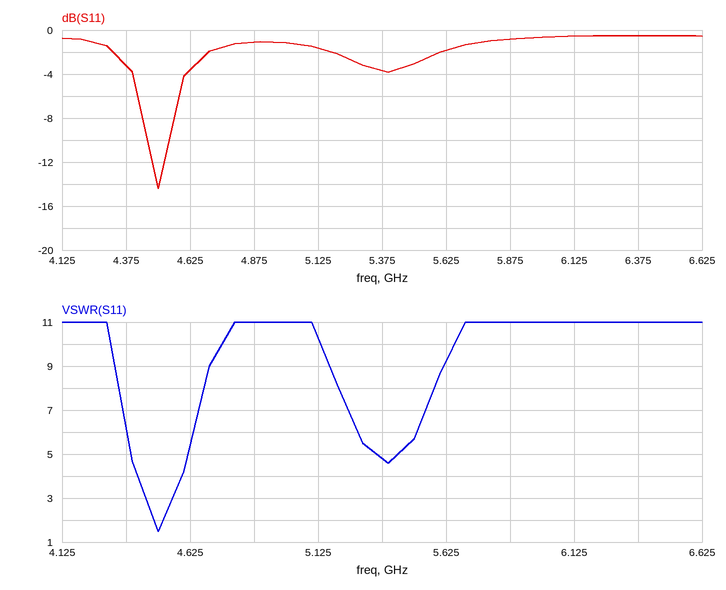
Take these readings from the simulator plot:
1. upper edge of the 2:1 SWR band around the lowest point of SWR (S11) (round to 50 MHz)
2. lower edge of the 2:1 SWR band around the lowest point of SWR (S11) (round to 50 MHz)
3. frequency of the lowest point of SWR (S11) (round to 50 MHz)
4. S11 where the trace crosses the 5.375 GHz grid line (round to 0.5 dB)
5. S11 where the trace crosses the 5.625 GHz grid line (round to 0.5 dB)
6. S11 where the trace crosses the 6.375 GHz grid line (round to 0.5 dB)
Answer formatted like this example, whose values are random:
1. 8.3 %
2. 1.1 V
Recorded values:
1. 4.50 GHz
2. 4.50 GHz
3. 4.50 GHz
4. -3.5 dB
5. -2.0 dB
6. -0.5 dB
